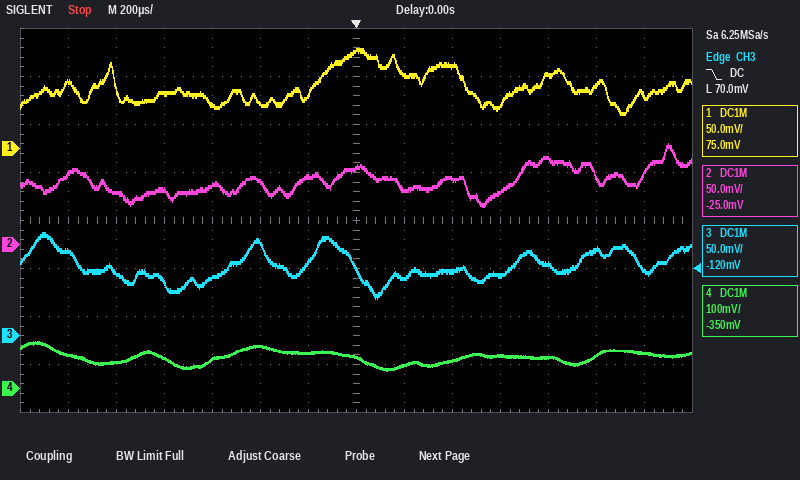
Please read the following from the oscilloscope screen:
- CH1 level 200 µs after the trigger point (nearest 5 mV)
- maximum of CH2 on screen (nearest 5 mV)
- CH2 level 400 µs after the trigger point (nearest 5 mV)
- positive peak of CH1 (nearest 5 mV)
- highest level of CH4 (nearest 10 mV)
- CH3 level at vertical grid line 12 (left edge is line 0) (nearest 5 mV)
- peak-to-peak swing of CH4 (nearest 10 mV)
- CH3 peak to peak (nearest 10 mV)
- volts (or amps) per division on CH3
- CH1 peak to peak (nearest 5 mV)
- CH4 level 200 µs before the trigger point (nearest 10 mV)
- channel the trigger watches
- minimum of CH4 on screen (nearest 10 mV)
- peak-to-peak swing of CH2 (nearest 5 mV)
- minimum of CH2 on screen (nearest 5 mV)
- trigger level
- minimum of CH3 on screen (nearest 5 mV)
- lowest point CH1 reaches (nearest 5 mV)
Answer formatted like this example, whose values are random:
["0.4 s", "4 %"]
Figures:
["75 mV", "105 mV", "70 mV", "105 mV", "100 mV", "90 mV", "60 mV", "70 mV", "50 mV", "70 mV", "70 mV", "CH3", "40 mV", "65 mV", "40 mV", "70.0 mV", "40 mV", "35 mV"]
